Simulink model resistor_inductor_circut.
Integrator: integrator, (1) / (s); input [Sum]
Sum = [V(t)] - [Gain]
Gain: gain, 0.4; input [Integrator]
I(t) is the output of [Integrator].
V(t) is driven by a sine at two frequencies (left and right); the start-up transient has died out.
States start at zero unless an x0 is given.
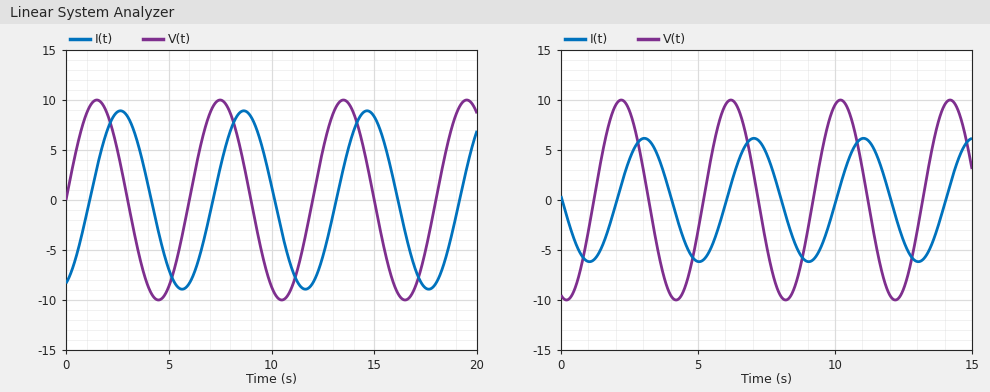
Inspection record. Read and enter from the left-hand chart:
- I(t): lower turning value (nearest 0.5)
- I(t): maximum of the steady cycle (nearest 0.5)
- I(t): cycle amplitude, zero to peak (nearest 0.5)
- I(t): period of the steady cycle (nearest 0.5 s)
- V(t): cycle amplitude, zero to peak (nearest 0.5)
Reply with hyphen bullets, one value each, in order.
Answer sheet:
- -9.0
- 9.0
- 9.0
- 6.0 s
- 10.0
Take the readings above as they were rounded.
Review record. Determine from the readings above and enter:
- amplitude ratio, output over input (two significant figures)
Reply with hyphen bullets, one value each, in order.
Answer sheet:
- 0.90
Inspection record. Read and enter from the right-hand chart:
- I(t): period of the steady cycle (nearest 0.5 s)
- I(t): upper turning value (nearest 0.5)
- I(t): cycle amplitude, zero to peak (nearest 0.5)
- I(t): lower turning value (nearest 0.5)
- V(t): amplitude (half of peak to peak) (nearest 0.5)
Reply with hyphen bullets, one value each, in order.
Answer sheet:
- 4.0 s
- 6.0
- 6.0
- -6.0
- 10.0
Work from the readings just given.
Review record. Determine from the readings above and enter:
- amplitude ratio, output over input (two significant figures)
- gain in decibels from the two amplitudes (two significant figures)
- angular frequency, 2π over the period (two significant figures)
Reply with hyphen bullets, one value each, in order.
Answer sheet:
- 0.60
- -4.4 dB
- 1.6 rad/s
